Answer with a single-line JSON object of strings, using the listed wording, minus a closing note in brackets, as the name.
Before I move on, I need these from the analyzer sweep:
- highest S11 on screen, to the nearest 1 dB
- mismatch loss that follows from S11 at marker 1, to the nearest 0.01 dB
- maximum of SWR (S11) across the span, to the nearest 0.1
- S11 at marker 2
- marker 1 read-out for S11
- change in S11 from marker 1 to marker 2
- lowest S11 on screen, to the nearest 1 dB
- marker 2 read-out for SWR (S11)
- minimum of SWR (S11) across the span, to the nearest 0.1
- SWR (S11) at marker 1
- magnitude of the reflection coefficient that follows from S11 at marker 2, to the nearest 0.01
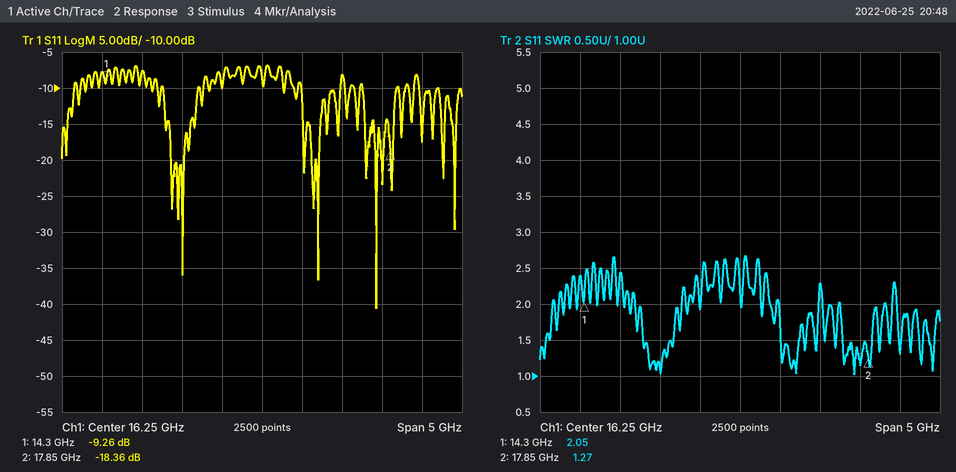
{"highest S11 on screen, to the nearest 1 dB": "-7 dB", "mismatch loss that follows from S11 at marker 1, to the nearest 0.01 dB": "0.55 dB", "maximum of SWR (S11) across the span, to the nearest 0.1": "2.7", "S11 at marker 2": "-18.36 dB", "marker 1 read-out for S11": "-9.26 dB", "change in S11 from marker 1 to marker 2": "-9.10 dB", "lowest S11 on screen, to the nearest 1 dB": "-41 dB", "marker 2 read-out for SWR": "1.27", "minimum of SWR (S11) across the span, to the nearest 0.1": "1.0", "SWR (S11) at marker 1": "2.05", "magnitude of the reflection coefficient that follows from S11 at marker 2, to the nearest 0.01": "0.12"}
